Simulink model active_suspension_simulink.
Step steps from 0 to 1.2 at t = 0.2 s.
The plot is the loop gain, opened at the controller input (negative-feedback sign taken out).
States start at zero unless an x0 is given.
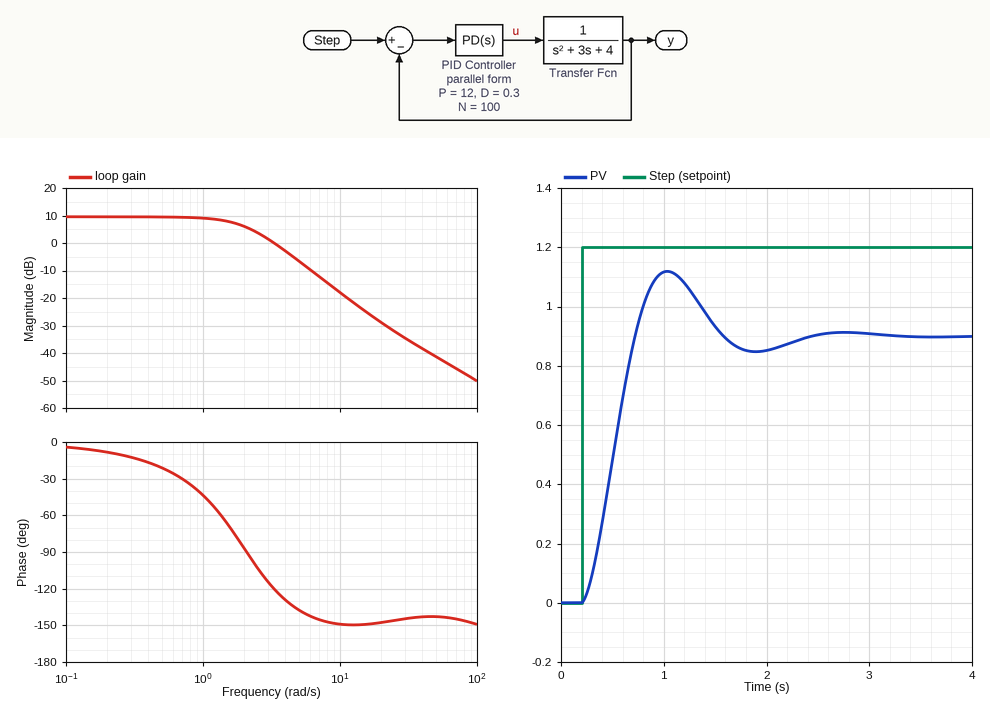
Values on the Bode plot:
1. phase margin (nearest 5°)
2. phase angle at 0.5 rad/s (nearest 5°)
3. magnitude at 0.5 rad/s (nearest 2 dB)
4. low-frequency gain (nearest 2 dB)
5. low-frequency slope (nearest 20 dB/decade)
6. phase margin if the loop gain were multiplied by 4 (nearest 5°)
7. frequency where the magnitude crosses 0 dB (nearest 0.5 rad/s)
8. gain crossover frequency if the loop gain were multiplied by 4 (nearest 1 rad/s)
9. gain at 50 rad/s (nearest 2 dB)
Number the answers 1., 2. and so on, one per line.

1. 60°
2. -20°
3. 10 dB
4. 10 dB
5. 0 dB/decade
6. 35°
7. 3.5 rad/s
8. 7 rad/s
9. -42 dB
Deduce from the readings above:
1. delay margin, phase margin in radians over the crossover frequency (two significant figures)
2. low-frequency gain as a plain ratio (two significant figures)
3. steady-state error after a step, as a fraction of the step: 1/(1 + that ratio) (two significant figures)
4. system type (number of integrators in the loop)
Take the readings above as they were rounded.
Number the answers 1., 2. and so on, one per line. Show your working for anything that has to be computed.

1. 60 × π / 180 / 3.5 = 0.30 s
2. 10^(10 / 20) = 3.2
3. 1 / (1 + 3.2) = 0.24
4. 0
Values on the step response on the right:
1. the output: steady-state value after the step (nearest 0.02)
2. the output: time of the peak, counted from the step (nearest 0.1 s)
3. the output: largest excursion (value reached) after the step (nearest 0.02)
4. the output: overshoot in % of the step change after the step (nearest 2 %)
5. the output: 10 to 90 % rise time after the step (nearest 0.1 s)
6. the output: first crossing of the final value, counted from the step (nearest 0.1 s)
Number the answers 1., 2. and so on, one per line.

1. 0.90
2. 0.8 s
3. 1.12
4. 24 %
5. 0.4 s
6. 0.5 s
